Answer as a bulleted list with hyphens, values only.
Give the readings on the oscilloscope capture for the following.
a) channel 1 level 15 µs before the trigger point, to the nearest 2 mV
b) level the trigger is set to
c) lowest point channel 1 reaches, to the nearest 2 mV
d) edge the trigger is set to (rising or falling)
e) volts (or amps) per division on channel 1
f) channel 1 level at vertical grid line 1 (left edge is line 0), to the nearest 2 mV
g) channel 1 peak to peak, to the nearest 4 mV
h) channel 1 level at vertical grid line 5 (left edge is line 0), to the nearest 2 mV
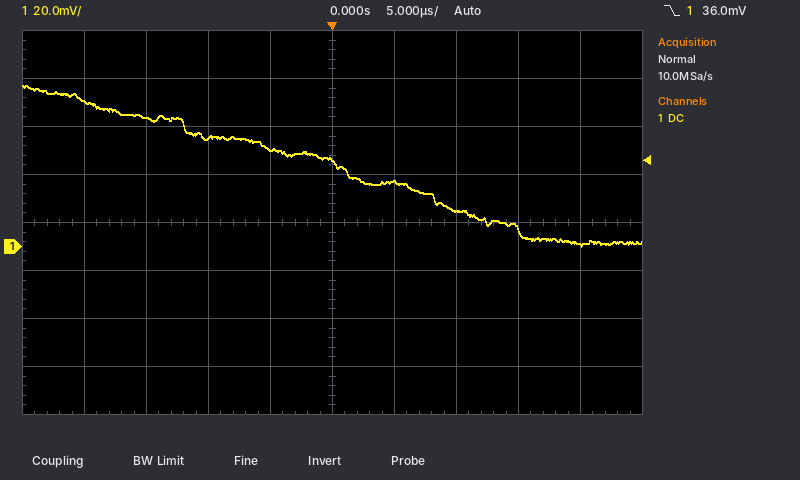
- 54 mV
- 36.0 mV
- 0 mV
- falling
- 20 mV
- 60 mV
- 68 mV
- 36 mV
